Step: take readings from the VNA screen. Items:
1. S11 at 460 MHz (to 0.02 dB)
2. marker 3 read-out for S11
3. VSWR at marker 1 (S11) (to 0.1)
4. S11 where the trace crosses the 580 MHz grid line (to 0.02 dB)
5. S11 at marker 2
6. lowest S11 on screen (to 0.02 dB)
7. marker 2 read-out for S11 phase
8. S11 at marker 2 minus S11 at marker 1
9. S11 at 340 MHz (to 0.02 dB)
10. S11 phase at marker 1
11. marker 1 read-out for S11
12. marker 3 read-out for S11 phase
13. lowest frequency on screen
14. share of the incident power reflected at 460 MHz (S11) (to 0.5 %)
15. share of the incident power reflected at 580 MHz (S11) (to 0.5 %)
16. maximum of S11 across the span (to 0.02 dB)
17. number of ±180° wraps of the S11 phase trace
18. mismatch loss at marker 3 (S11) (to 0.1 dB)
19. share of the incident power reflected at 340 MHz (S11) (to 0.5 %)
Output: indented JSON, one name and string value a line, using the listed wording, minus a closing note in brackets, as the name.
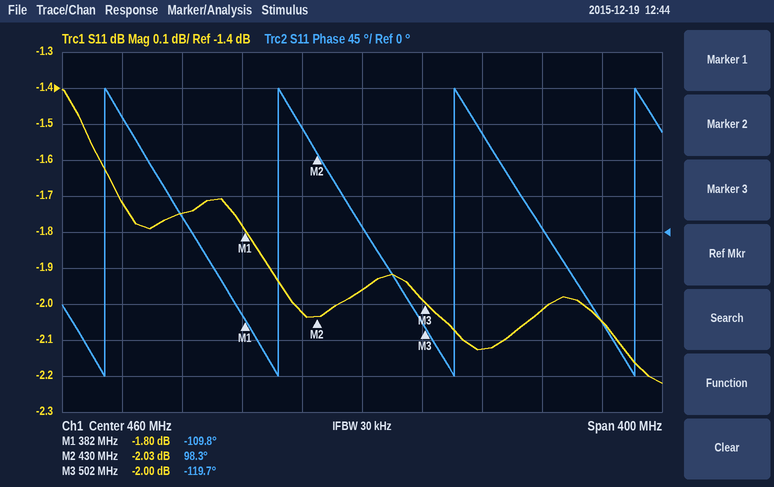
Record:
{
  "S11 at 460 MHz": "-1.96 dB",
  "marker 3 read-out for S11": "-2.00 dB",
  "VSWR at marker 1 (S11)": "9.7",
  "S11 where the trace crosses the 580 MHz grid line": "-2.02 dB",
  "S11 at marker 2": "-2.03 dB",
  "lowest S11 on screen": "-2.22 dB",
  "marker 2 read-out for S11 phase": "98.3°",
  "S11 at marker 2 minus S11 at marker 1": "-0.23 dB",
  "S11 at 340 MHz": "-1.74 dB",
  "S11 phase at marker 1": "-109.8°",
  "marker 1 read-out for S11": "-1.80 dB",
  "marker 3 read-out for S11 phase": "-119.7°",
  "lowest frequency on screen": "260 MHz",
  "share of the incident power reflected at 460 MHz (S11)": "63.5 %",
  "share of the incident power reflected at 580 MHz (S11)": "63.0 %",
  "maximum of S11 across the span": "-1.40 dB",
  "number of ±180° wraps of the S11 phase trace": "4",
  "mismatch loss at marker 3 (S11)": "4.3 dB",
  "share of the incident power reflected at 340 MHz (S11)": "67.0 %"
}
